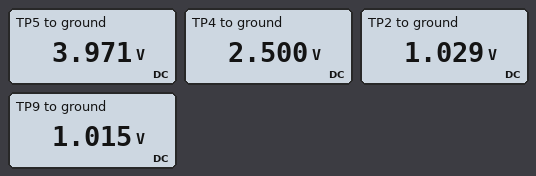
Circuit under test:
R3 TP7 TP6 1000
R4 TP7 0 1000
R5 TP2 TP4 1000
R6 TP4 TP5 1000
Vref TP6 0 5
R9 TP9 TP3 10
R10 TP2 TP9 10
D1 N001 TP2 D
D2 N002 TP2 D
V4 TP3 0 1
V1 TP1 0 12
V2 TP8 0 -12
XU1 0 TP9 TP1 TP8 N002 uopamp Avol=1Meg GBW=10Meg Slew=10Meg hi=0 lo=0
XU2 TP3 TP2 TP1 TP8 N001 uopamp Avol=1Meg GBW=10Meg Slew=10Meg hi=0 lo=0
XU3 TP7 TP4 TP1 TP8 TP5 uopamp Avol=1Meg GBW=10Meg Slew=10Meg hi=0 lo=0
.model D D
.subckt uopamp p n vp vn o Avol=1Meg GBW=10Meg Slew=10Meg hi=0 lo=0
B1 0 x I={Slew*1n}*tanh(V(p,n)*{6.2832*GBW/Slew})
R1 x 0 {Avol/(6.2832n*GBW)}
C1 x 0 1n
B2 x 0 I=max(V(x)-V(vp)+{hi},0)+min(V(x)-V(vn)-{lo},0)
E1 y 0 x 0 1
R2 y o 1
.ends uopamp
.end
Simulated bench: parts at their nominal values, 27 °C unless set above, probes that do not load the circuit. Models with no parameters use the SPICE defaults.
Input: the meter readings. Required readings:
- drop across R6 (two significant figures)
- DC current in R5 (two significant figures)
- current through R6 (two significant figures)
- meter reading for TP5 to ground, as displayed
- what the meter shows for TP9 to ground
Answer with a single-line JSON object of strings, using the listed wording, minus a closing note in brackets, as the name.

{"drop across R6": "1.5 V", "DC current in R5": "1.5 mA", "current through R6": "1.5 mA", "meter reading for TP5 to ground, as displayed": "3.971 V", "what the meter shows for TP9 to ground": "1.015 V"}
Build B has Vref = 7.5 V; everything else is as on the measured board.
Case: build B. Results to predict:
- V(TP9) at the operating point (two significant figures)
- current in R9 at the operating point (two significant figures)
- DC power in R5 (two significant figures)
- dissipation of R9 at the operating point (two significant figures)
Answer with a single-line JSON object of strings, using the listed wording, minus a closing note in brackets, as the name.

{"V(TP9) at the operating point": "1.0 V", "current in R9 at the operating point": "2.7 mA", "DC power in R5": "7.3 mW", "dissipation of R9 at the operating point": "73 µW"}
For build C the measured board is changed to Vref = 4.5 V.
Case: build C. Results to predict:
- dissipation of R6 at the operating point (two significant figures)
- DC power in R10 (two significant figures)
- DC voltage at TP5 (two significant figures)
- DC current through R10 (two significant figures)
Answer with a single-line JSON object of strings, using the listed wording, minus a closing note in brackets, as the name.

{"dissipation of R6 at the operating point": "1.5 mW", "DC power in R10": "15 µW", "DC voltage at TP5": "3.5 V", "DC current through R10": "1.2 mA"}
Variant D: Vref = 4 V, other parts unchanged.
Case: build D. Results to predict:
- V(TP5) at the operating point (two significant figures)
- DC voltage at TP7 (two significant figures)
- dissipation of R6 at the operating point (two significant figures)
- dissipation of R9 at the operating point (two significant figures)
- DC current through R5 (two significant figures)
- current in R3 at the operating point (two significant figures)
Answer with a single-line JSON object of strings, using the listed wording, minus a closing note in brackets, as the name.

{"V(TP5) at the operating point": "3.0 V", "DC voltage at TP7": "2.0 V", "dissipation of R6 at the operating point": "960 µW", "dissipation of R9 at the operating point": "9.6 µW", "DC current through R5": "980 µA", "current in R3 at the operating point": "2.0 mA"}
